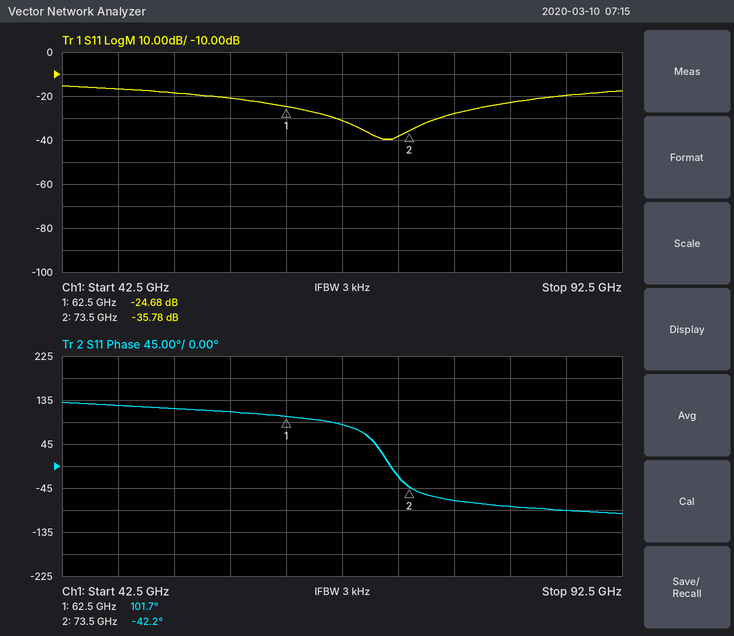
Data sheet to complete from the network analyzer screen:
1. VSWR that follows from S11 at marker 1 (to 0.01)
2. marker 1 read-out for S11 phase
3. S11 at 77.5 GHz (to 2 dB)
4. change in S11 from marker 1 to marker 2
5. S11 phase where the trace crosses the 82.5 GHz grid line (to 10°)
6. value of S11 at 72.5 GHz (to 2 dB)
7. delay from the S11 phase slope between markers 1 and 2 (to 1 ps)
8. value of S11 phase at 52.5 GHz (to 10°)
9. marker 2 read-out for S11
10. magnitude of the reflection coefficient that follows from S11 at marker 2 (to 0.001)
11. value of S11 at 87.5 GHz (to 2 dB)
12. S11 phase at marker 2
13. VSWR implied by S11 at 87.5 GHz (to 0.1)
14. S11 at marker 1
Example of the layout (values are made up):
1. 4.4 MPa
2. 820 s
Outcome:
1. 1.12
2. 101.7°
3. -28 dB
4. -11.10 dB
5. -80°
6. -38 dB
7. 36 ps
8. 120°
9. -35.78 dB
10. 0.016
11. -20 dB
12. -42.2°
13. 1.2
14. -24.68 dB
